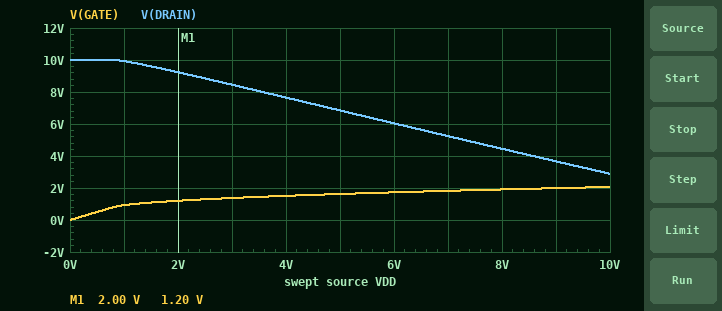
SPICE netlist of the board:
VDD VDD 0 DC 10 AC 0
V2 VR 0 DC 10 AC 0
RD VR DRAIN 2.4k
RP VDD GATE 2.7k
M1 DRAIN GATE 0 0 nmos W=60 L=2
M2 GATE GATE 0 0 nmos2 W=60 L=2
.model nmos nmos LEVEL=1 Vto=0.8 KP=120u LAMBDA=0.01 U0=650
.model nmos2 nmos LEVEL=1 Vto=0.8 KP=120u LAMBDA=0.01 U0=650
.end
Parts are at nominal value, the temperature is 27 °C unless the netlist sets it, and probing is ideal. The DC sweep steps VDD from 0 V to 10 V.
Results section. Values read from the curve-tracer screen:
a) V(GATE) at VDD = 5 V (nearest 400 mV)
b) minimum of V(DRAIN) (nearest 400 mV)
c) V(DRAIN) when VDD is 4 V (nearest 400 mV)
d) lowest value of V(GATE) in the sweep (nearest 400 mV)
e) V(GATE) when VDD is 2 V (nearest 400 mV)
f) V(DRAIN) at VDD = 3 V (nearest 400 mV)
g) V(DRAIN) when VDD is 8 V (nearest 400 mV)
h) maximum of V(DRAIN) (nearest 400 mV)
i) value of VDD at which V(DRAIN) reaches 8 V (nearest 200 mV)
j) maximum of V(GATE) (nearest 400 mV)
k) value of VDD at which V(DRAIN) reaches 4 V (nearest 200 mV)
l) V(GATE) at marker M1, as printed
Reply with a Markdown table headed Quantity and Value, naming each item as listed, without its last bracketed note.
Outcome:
| Quantity | Value |
|---|---|
| V(GATE) at VDD = 5 V | 1.6 V |
| minimum of V(DRAIN) | 2.8 V |
| V(DRAIN) when VDD is 4 V | 7.6 V |
| lowest value of V(GATE) in the sweep | 0 V |
| V(GATE) when VDD is 2 V | 1.2 V |
| V(DRAIN) at VDD = 3 V | 8.4 V |
| V(DRAIN) when VDD is 8 V | 4.4 V |
| maximum of V(DRAIN) | 10.0 V |
| value of VDD at which V(DRAIN) reaches 8 V | 3.6 V |
| maximum of V(GATE) | 2.0 V |
| value of VDD at which V(DRAIN) reaches 4 V | 8.6 V |
| V(GATE) at marker M1, as printed | 1.20 V |
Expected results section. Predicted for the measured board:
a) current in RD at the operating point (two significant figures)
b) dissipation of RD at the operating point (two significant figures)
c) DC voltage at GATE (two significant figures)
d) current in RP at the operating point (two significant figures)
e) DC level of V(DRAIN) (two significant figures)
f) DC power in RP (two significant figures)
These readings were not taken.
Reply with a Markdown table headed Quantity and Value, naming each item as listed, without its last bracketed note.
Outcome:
| Quantity | Value |
|---|---|
| current in RD at the operating point | 3.0 mA |
| dissipation of RD at the operating point | 21 mW |
| DC voltage at GATE | 2.1 V |
| current in RP at the operating point | 2.9 mA |
| DC level of V(DRAIN) | 2.9 V |
| DC power in RP | 23 mW |
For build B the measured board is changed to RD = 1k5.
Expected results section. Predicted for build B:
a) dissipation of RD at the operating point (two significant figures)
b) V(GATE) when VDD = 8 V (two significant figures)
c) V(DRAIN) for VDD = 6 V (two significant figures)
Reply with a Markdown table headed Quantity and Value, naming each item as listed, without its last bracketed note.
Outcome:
| Quantity | Value |
|---|---|
| dissipation of RD at the operating point | 14 mW |
| V(GATE) when VDD = 8 V | 1.9 V |
| V(DRAIN) for VDD = 6 V | 7.5 V |
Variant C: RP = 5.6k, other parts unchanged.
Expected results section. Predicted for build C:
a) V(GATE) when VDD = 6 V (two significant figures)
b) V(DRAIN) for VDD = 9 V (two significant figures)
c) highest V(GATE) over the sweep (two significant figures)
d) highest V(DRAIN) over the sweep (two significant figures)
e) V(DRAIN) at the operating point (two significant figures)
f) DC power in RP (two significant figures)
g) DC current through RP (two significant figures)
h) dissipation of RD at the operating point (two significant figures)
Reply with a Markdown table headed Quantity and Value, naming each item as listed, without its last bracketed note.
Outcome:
| Quantity | Value |
|---|---|
| V(GATE) when VDD = 6 V | 1.5 V |
| V(DRAIN) for VDD = 9 V | 6.7 V |
| highest V(GATE) over the sweep | 1.7 V |
| highest V(DRAIN) over the sweep | 10 V |
| V(DRAIN) at the operating point | 6.3 V |
| DC power in RP | 12 mW |
| DC current through RP | 1.5 mA |
| dissipation of RD at the operating point | 5.8 mW |
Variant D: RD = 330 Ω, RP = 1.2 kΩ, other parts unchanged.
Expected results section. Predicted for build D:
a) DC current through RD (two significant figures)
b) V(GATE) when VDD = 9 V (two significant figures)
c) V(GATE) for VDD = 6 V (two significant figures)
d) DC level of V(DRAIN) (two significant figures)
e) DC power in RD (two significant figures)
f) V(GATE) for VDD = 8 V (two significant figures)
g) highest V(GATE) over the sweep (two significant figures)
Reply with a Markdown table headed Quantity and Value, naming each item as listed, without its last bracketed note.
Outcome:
| Quantity | Value |
|---|---|
| DC current through RD | 6.5 mA |
| V(GATE) when VDD = 9 V | 2.5 V |
| V(GATE) for VDD = 6 V | 2.1 V |
| DC level of V(DRAIN) | 7.9 V |
| DC power in RD | 14 mW |
| V(GATE) for VDD = 8 V | 2.4 V |
| highest V(GATE) over the sweep | 2.6 V |
